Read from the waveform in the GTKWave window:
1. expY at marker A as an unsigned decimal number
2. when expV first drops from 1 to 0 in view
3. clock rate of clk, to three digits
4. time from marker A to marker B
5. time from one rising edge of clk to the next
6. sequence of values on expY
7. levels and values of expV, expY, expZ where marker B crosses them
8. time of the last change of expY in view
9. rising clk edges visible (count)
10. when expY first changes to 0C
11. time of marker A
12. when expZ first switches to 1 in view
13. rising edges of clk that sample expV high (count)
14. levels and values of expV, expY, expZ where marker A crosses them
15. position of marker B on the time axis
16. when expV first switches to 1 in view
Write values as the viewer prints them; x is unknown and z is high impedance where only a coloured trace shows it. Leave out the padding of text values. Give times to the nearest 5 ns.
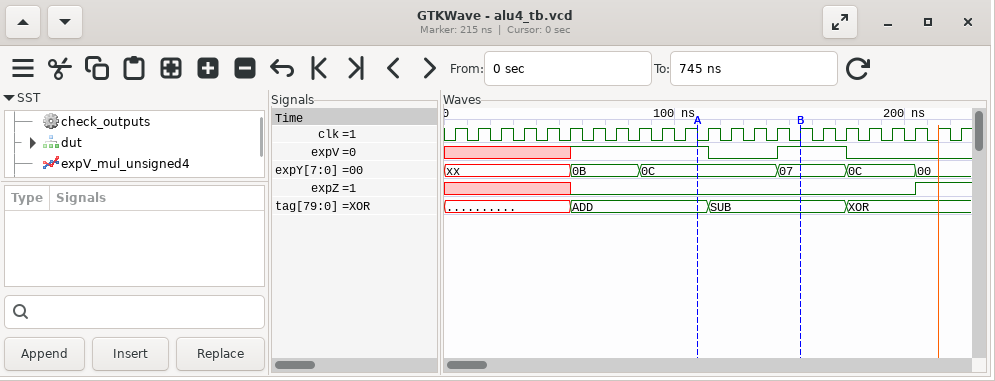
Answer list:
12
115 ns
100 MHz
45 ns
10 ns
xx, 0B, 0C, 07, 0C, 00
expV=1, expY=07, expZ=0
205 ns
23
85 ns
110 ns
205 ns
9
expV=1, expY=0C, expZ=0
155 ns
55 ns
